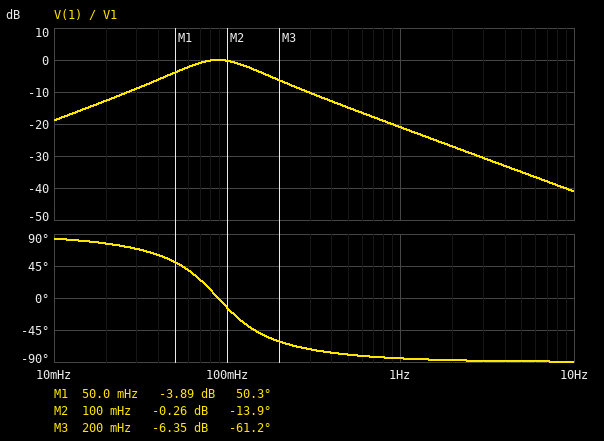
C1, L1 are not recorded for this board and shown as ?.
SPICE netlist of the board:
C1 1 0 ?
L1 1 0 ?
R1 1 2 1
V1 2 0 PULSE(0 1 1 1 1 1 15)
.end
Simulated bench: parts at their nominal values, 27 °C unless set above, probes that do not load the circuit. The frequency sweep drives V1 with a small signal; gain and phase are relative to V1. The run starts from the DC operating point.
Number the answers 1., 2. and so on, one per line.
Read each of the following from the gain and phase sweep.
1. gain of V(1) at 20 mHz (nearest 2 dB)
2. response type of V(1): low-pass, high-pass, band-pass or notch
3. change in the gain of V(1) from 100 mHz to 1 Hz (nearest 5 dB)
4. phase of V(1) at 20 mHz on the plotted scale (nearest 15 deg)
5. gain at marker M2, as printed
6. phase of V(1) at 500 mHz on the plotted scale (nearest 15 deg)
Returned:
1. -12 dB
2. band-pass
3. -20 dB
4. 75 deg
5. -0.26 dB
6. -75 deg
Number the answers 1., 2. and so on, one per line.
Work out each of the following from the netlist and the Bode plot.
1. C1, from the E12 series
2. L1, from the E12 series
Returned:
1. 1.8 F
2. 1.8 H
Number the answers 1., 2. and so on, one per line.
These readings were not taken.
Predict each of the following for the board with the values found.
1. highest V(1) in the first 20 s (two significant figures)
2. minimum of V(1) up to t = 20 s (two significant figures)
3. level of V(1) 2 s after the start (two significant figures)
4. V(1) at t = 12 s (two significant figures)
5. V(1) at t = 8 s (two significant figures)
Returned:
1. 510 mV
2. -310 mV
3. 230 mV
4. 28 mV
5. -270 mV
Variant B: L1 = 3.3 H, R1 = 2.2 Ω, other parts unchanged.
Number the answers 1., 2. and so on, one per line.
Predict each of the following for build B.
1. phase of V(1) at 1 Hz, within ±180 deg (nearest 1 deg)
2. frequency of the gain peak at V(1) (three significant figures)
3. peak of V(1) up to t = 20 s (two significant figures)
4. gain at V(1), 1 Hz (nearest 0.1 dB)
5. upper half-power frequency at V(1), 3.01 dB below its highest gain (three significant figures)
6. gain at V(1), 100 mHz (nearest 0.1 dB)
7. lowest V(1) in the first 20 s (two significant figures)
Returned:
1. -88 deg
2. 65.3 mHz
3. 390 mV
4. -27.9 dB
5. 88.4 mHz
6. -4.8 dB
7. -220 mV
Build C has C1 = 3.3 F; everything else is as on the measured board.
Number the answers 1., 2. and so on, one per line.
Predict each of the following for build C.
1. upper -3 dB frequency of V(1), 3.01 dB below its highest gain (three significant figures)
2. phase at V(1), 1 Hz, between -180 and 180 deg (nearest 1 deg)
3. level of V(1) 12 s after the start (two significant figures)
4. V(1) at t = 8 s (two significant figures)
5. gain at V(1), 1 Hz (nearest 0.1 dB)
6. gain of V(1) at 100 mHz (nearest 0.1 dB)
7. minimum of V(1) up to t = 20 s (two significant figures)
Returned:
1. 93.7 mHz
2. -87 deg
3. -100 mV
4. -210 mV
5. -26.3 dB
6. -3.8 dB
7. -230 mV
